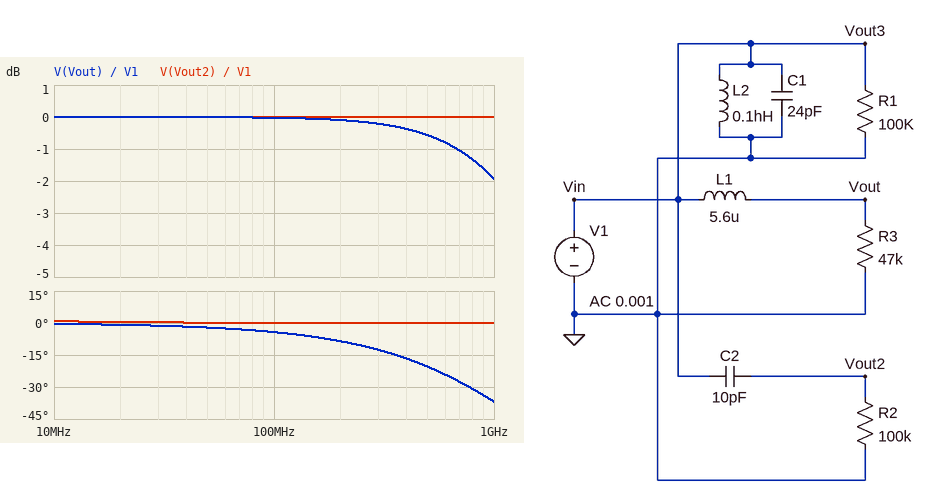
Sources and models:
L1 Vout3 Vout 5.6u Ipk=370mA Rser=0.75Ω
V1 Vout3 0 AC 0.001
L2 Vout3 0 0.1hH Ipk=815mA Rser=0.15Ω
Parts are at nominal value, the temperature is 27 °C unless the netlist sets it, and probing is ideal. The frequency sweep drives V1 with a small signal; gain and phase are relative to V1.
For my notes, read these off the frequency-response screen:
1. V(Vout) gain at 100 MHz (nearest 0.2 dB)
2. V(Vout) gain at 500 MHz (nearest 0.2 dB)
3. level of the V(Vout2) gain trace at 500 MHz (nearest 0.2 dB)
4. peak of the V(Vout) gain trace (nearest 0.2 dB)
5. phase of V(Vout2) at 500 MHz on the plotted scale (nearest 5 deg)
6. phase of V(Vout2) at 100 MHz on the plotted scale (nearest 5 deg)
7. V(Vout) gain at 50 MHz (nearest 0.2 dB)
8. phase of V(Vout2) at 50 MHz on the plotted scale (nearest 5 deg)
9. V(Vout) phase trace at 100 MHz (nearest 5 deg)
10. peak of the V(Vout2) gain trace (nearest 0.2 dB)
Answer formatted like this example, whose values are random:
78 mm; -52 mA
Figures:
0 dB; -0.6 dB; 0 dB; 0 dB; 0 deg; 0 deg; 0 dB; 0 deg; -5 deg; 0 dB
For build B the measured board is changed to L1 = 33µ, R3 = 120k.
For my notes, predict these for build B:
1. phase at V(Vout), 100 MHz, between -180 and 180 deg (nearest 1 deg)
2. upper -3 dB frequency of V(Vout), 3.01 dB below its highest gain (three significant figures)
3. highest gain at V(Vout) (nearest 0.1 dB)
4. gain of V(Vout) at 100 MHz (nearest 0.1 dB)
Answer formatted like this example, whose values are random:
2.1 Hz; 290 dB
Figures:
-10 deg; 579 MHz; 0 dB; -0.1 dB
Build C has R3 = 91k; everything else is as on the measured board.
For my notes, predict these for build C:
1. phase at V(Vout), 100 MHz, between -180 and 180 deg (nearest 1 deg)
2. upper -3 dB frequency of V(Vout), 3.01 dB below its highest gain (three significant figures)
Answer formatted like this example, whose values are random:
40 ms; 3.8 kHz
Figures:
-2 deg; 2.59 GHz
